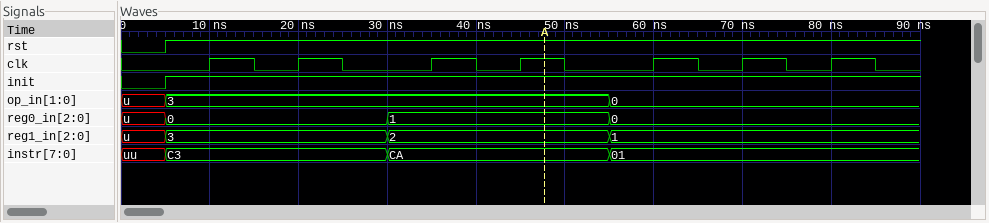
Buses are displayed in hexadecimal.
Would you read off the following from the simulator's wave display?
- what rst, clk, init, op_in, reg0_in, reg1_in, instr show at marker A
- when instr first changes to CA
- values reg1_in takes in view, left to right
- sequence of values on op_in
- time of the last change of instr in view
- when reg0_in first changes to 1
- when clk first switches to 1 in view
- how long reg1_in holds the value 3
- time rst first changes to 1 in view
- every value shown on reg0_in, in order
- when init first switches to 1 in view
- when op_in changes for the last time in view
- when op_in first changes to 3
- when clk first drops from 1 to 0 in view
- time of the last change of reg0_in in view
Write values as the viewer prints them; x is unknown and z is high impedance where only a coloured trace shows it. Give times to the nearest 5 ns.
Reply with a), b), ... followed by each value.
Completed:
a) rst=1, clk=1, init=1, op_in=3, reg0_in=1, reg1_in=2, instr=CA
b) 30 ns
c) u, 3, 2, 1
d) u, 3, 0
e) 55 ns
f) 30 ns
g) 10 ns
h) 25 ns
i) 5 ns
j) u, 0, 1, 0
k) 5 ns
l) 55 ns
m) 5 ns
n) 15 ns
o) 55 ns
